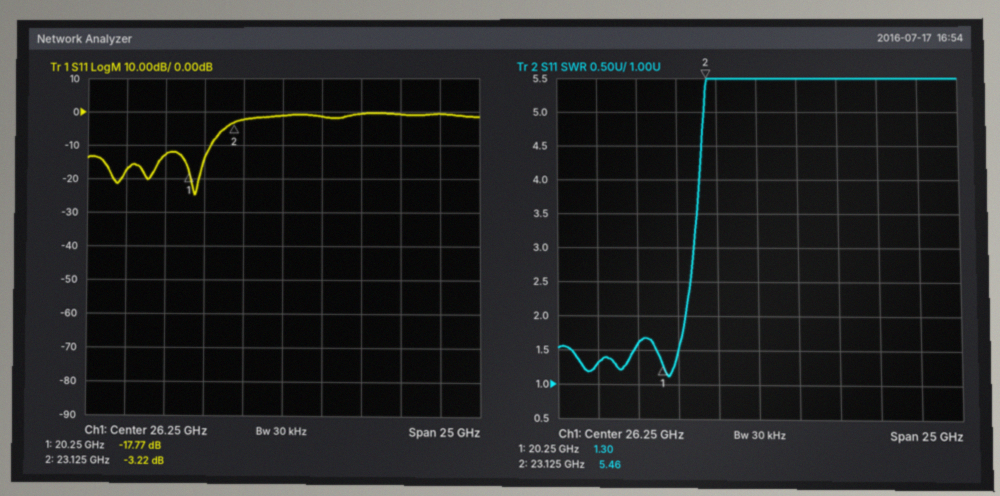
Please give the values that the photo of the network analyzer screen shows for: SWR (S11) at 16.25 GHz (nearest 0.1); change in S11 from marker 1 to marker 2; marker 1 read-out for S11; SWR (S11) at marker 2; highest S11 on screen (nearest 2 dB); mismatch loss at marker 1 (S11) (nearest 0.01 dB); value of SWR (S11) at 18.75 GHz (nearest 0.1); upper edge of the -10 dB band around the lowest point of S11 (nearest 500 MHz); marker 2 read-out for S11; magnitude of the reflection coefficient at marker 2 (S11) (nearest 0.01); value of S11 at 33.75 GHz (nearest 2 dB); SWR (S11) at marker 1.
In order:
1.3
14.55 dB
-17.77 dB
5.46
0 dB
0.07 dB
1.6
21.5 GHz
-3.22 dB
0.69
0 dB
1.30
